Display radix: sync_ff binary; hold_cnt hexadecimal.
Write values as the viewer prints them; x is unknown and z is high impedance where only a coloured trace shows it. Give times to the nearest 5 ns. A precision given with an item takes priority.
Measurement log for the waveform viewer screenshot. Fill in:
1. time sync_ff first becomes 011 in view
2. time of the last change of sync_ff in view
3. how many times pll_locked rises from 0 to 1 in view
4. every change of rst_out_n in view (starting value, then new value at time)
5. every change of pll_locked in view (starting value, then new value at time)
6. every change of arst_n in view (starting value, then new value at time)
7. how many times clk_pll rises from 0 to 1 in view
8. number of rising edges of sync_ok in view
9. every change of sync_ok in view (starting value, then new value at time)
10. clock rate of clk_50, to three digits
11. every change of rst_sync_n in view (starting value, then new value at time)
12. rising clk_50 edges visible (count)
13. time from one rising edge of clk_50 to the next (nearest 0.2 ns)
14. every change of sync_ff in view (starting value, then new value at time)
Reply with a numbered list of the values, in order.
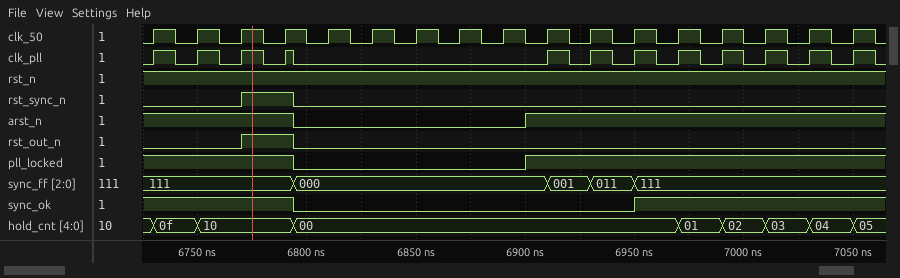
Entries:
1. 6930 ns
2. 6950 ns
3. 1
4. 0, 1 at 6770 ns, 0 at 6795 ns
5. 1, 0 at 6795 ns, 1 at 6900 ns
6. 1, 0 at 6795 ns, 1 at 6900 ns
7. 12
8. 1
9. 1, 0 at 6795 ns, 1 at 6950 ns
10. 50.0 MHz
11. 0, 1 at 6770 ns, 0 at 6795 ns
12. 17
13. 20 ns
14. 111, 000 at 6795 ns, 001 at 6910 ns, 011 at 6930 ns, 111 at 6950 ns
